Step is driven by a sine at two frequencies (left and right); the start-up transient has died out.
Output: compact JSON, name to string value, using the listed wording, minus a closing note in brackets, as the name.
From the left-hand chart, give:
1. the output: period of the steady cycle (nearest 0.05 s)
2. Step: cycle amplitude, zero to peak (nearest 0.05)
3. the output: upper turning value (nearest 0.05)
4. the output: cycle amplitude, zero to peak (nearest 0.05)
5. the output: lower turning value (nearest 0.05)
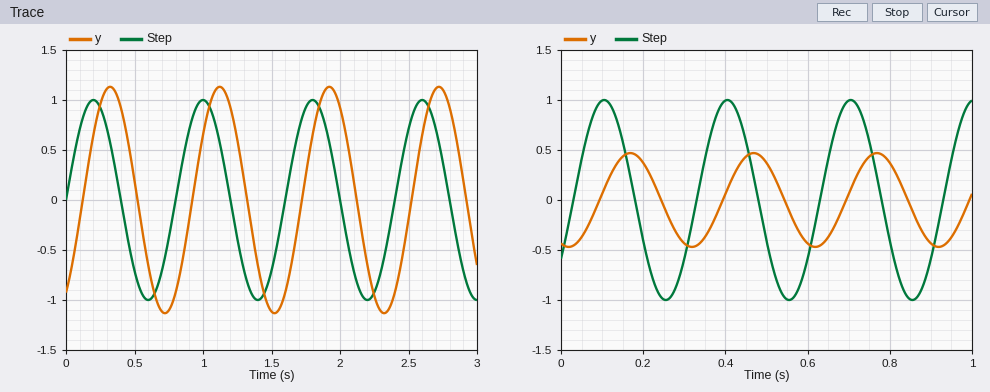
{"the output: period of the steady cycle": "0.80 s", "Step: cycle amplitude, zero to peak": "1.00", "the output: upper turning value": "1.15", "the output: cycle amplitude, zero to peak": "1.15", "the output: lower turning value": "-1.15"}
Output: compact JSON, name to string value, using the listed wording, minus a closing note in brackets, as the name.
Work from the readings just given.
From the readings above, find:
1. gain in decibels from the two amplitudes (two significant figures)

{"gain in decibels from the two amplitudes": "1.2 dB"}
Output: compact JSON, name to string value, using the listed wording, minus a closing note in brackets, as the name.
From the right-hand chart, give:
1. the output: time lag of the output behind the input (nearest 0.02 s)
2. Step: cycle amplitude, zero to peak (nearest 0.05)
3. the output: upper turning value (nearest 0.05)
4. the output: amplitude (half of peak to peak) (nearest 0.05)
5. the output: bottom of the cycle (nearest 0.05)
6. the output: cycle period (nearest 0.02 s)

{"the output: time lag of the output behind the input": "0.06 s", "Step: cycle amplitude, zero to peak": "1.00", "the output: upper turning value": "0.45", "the output: amplitude (half of peak to peak)": "0.45", "the output: bottom of the cycle": "-0.45", "the output: cycle period": "0.30 s"}
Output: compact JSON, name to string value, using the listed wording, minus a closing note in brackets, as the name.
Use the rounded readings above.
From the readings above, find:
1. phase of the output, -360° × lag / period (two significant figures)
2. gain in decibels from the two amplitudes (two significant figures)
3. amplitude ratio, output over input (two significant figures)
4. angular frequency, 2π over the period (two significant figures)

{"phase of the output, -360° × lag / period": "-72°", "gain in decibels from the two amplitudes": "-6.9 dB", "amplitude ratio, output over input": "0.45", "angular frequency, 2π over the period": "21 rad/s"}
